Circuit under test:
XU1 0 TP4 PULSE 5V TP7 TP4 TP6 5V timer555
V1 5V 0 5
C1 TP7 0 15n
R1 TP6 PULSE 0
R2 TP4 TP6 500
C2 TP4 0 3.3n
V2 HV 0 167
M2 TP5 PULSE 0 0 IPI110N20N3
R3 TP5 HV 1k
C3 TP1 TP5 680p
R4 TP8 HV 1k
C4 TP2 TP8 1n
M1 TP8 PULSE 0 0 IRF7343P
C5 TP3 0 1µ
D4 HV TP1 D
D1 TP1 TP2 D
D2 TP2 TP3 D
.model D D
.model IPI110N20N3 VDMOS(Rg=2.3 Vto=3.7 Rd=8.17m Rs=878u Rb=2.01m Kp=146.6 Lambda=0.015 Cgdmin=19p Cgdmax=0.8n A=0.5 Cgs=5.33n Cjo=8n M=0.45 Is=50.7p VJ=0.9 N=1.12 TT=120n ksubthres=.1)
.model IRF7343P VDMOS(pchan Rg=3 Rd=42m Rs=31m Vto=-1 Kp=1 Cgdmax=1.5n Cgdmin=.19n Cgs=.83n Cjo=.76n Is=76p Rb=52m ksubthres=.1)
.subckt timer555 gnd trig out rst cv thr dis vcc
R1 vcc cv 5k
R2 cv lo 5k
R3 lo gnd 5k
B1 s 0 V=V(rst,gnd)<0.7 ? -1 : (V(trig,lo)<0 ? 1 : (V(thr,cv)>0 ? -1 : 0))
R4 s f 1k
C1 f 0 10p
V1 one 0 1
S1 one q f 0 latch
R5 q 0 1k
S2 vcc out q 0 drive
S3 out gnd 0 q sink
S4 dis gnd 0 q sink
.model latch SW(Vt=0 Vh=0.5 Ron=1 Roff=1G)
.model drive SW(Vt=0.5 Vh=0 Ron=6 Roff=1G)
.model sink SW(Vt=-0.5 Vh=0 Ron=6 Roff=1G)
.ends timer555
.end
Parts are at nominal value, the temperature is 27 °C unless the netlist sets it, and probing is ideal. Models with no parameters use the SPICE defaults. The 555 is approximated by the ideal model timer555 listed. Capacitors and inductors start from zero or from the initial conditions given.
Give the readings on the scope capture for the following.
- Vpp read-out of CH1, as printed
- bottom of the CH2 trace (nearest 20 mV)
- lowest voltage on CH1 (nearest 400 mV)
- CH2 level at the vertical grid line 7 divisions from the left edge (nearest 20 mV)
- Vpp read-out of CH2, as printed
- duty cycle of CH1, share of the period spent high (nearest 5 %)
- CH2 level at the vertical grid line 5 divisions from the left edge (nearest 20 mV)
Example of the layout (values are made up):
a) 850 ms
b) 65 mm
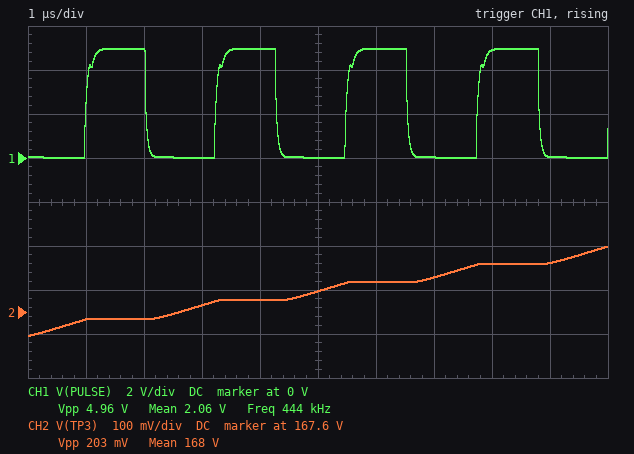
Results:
a) 4.96 V
b) 167.54 V
c) 0 V
d) 167.68 V
e) 203 mV
f) 45 %
g) 167.64 V
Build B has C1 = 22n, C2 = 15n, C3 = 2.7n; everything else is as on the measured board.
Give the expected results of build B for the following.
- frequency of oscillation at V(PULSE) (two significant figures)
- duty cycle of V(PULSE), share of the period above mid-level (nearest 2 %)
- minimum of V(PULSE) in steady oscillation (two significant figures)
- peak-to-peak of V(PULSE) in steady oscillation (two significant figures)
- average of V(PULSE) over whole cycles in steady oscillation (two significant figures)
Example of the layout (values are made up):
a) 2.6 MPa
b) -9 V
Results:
a) 110 kHz
b) 42 %
c) 9.1 mV
d) 5.0 V
e) 2.1 V
